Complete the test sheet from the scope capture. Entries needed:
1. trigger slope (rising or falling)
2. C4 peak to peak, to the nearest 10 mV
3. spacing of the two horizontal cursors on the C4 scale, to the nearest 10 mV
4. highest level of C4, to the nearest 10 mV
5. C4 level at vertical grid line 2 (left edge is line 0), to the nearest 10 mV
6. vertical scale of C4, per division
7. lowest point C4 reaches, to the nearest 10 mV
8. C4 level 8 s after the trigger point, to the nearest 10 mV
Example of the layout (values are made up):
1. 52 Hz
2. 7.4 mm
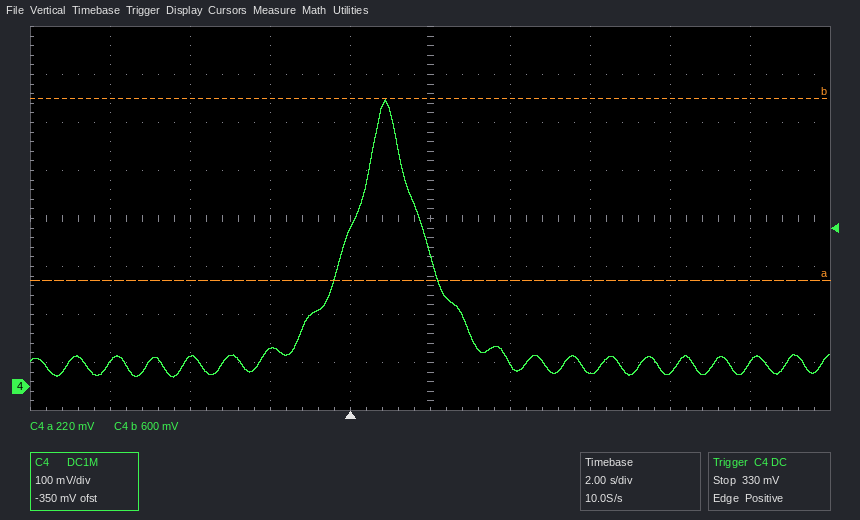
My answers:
1. rising
2. 580 mV
3. 380 mV
4. 600 mV
5. 60 mV
6. 100 mV
7. 20 mV
8. 30 mV
